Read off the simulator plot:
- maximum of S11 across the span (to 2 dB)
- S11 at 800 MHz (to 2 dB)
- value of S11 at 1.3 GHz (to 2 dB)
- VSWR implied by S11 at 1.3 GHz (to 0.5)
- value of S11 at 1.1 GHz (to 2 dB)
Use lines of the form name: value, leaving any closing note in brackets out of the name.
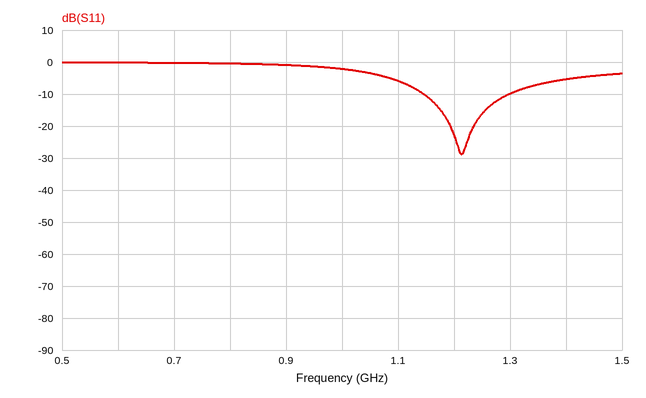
maximum of S11 across the span: 0 dB
S11 at 800 MHz: 0 dB
value of S11 at 1.3 GHz: -10 dB
VSWR implied by S11 at 1.3 GHz: 2.0
value of S11 at 1.1 GHz: -6 dB
